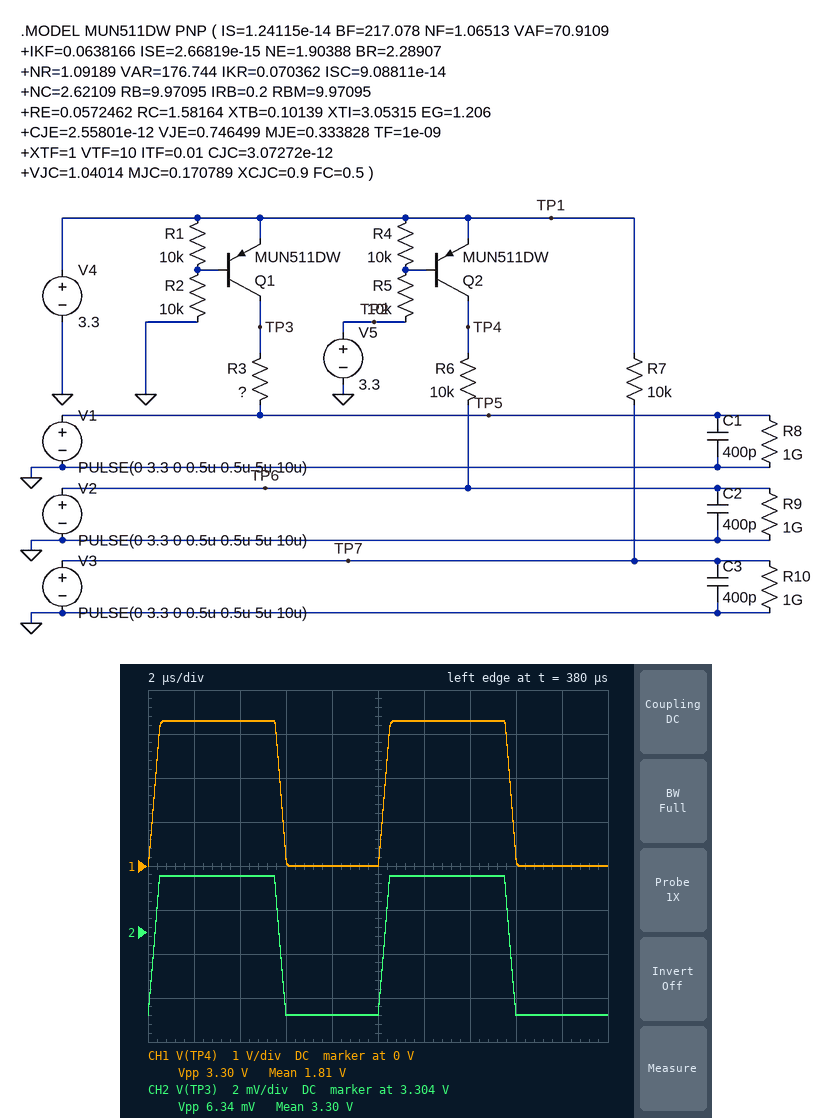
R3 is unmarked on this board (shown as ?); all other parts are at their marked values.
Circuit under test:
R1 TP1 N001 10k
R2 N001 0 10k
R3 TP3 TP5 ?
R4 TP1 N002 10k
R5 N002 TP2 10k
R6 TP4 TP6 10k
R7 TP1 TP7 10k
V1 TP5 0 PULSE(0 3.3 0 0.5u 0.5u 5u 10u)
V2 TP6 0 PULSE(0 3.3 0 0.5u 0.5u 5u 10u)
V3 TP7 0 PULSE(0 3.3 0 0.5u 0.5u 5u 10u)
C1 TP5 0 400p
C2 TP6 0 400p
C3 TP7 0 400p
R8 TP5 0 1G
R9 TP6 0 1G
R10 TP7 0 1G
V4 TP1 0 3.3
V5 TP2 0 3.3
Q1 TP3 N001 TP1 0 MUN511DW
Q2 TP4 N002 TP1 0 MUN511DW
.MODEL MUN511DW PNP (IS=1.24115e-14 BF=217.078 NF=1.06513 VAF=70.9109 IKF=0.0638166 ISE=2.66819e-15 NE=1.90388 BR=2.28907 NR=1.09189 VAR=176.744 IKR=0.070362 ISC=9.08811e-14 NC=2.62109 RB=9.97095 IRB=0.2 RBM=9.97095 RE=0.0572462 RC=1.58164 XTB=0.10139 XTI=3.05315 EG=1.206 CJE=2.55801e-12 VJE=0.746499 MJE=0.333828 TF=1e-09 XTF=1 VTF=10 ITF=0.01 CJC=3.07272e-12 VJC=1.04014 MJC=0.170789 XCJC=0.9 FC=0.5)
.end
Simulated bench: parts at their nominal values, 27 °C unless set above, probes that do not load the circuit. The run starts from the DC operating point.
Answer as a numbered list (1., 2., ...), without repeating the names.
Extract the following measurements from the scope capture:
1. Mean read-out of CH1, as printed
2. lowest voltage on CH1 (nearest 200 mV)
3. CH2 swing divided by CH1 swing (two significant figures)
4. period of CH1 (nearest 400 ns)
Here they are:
1. 1.81 V
2. 0 V
3. 0.0019
4. 10.0 µs
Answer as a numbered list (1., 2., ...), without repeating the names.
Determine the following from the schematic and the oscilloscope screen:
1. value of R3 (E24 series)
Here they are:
1. 22 kΩ
